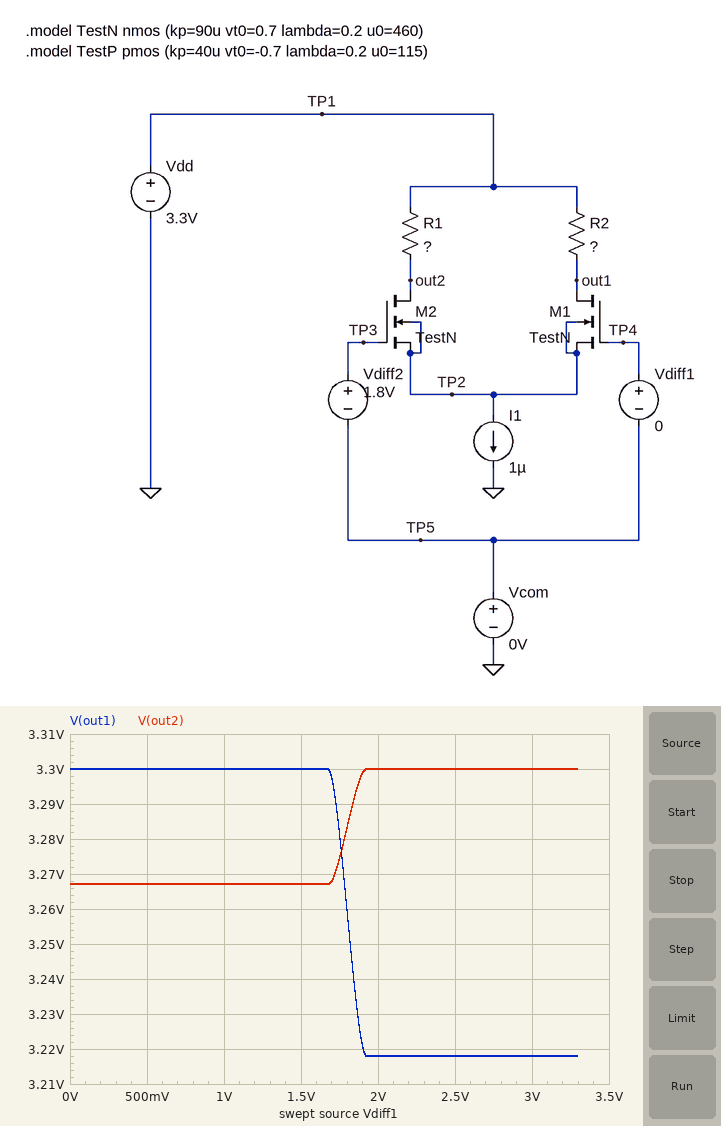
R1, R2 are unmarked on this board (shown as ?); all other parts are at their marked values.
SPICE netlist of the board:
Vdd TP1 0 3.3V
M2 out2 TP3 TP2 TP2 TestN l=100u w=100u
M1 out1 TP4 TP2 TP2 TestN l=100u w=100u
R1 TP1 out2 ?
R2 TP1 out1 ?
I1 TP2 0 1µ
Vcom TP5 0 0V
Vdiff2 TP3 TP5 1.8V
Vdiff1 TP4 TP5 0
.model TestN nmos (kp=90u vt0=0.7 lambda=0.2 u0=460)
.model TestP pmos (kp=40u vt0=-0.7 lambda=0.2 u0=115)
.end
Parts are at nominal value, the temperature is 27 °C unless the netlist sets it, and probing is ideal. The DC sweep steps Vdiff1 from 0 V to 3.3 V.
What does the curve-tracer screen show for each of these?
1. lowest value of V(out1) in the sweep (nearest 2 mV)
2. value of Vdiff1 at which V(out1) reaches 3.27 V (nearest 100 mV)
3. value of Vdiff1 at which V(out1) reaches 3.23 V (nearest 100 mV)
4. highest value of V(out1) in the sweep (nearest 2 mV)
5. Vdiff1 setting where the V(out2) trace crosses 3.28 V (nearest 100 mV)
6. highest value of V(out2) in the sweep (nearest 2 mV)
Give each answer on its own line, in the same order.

3.218 V
1.8 V
1.9 V
3.300 V
1.8 V
3.300 V
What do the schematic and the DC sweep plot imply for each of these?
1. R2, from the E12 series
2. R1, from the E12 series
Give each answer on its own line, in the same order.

82 kΩ
33 kΩ
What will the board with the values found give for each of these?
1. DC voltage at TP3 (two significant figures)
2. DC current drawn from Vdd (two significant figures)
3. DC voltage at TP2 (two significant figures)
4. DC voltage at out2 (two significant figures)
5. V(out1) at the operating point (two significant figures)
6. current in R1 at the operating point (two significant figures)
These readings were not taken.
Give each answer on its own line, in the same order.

1.8 V
1.0 µA
980 mV
3.3 V
3.3 V
1.0 µA
